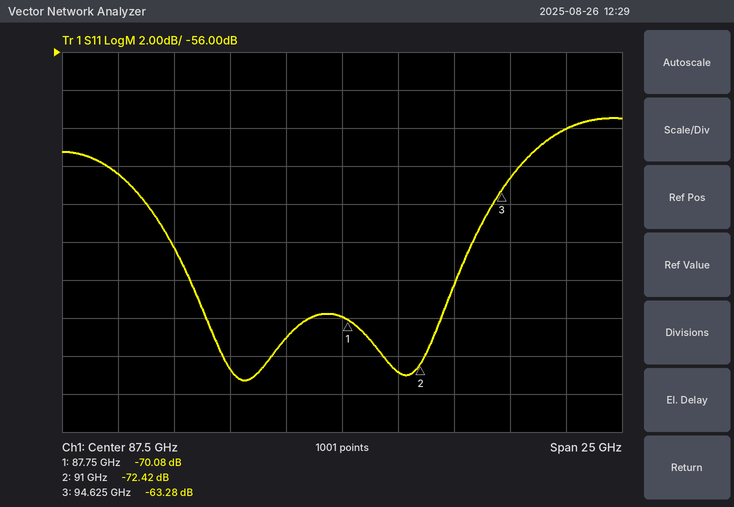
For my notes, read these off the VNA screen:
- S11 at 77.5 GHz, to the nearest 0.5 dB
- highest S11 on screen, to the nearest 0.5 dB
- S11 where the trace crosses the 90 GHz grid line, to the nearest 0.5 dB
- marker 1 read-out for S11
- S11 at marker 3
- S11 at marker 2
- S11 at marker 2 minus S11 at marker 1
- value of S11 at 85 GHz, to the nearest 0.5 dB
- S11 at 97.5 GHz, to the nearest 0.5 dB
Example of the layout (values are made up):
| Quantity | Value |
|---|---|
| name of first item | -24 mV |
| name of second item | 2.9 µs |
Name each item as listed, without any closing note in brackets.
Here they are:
| Quantity | Value |
|---|---|
| S11 at 77.5 GHz, to the nearest 0.5 dB | -62.5 dB |
| highest S11 on screen, to the nearest 0.5 dB | -59.5 dB |
| S11 where the trace crosses the 90 GHz grid line, to the nearest 0.5 dB | -73.0 dB |
| marker 1 read-out for S11 | -70.08 dB |
| S11 at marker 3 | -63.28 dB |
| S11 at marker 2 | -72.42 dB |
| S11 at marker 2 minus S11 at marker 1 | -2.34 dB |
| value of S11 at 85 GHz, to the nearest 0.5 dB | -71.0 dB |
| S11 at 97.5 GHz, to the nearest 0.5 dB | -60.0 dB |
